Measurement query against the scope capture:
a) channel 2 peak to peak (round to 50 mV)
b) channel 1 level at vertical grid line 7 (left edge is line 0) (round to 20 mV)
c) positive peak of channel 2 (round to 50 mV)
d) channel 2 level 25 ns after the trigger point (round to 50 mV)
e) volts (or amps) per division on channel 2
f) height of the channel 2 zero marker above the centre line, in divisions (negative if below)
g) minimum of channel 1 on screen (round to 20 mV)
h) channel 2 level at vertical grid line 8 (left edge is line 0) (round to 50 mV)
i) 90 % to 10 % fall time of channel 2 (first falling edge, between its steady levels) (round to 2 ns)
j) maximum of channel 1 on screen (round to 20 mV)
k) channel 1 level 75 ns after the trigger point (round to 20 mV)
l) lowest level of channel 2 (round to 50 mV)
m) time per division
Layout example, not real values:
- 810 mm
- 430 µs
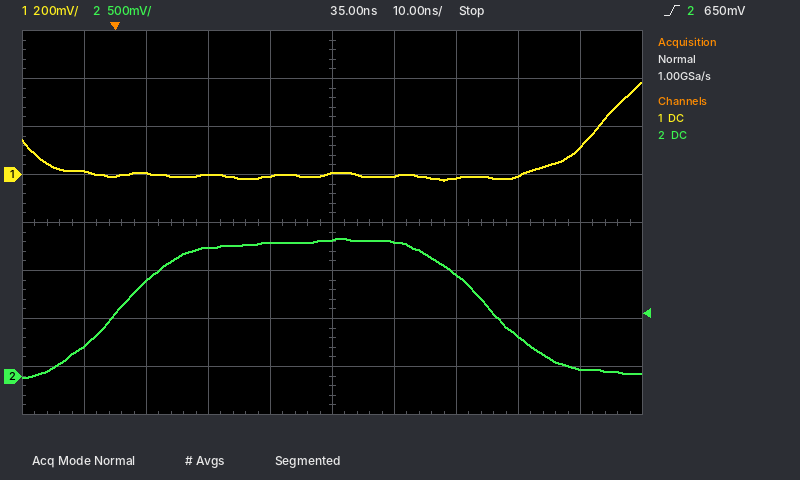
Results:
- 1.45 V
- -20 mV
- 1.45 V
- 1.40 V
- 500 mV
- -3.2 div
- -20 mV
- 400 mV
- 20 ns
- 380 mV
- 120 mV
- 0 mV
- 10 ns
